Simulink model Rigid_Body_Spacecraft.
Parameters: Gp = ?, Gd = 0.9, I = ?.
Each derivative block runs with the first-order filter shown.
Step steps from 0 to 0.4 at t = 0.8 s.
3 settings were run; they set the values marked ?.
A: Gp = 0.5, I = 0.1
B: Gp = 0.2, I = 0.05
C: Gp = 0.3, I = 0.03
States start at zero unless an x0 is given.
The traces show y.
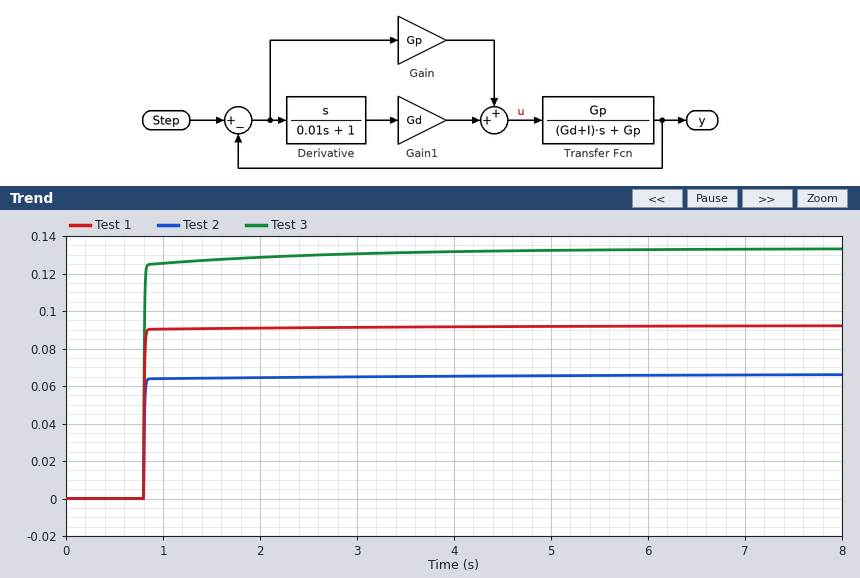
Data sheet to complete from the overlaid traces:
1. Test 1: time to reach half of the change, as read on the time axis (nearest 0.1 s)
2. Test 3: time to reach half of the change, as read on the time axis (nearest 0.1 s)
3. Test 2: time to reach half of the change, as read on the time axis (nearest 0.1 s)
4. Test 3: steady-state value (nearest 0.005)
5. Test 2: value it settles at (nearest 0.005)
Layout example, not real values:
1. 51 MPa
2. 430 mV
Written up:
1. 0.8 s
2. 0.8 s
3. 0.8 s
4. 0.135
5. 0.065
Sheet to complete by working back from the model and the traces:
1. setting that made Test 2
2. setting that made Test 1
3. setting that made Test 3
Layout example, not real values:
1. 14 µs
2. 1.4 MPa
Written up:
1. B
2. C
3. A
